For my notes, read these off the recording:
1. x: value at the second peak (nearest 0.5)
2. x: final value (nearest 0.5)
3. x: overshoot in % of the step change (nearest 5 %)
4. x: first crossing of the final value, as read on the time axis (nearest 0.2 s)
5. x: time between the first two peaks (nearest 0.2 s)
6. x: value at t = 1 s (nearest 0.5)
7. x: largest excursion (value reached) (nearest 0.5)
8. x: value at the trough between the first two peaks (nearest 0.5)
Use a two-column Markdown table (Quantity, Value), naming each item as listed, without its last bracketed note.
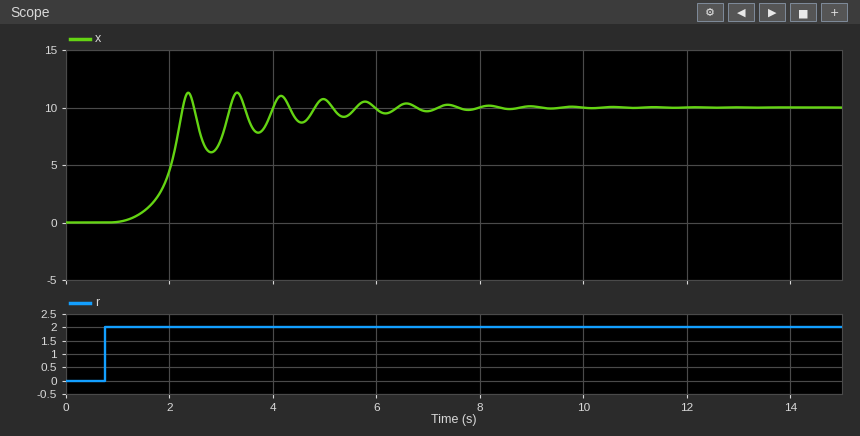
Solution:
| Quantity | Value |
|---|---|
| x: value at the second peak | 11.5 |
| x: final value | 10.0 |
| x: overshoot in % of the step change | 15 % |
| x: first crossing of the final value, as read on the time axis | 2.2 s |
| x: time between the first two peaks | 1.0 s |
| x: value at t = 1 s | 0.0 |
| x: largest excursion (value reached) | 11.5 |
| x: value at the trough between the first two peaks | 6.0 |
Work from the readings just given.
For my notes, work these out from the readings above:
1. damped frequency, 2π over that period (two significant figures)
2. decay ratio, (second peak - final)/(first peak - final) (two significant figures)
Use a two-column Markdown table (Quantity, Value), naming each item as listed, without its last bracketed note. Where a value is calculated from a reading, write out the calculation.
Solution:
| Quantity | Value |
|---|---|
| damped frequency, 2π over that period | 2π / 1 = 6.3 rad/s |
| decay ratio, (second peak - final)/(first peak - final) | (11.5 - 10) / (11.5 - 10) = 1.0 |
